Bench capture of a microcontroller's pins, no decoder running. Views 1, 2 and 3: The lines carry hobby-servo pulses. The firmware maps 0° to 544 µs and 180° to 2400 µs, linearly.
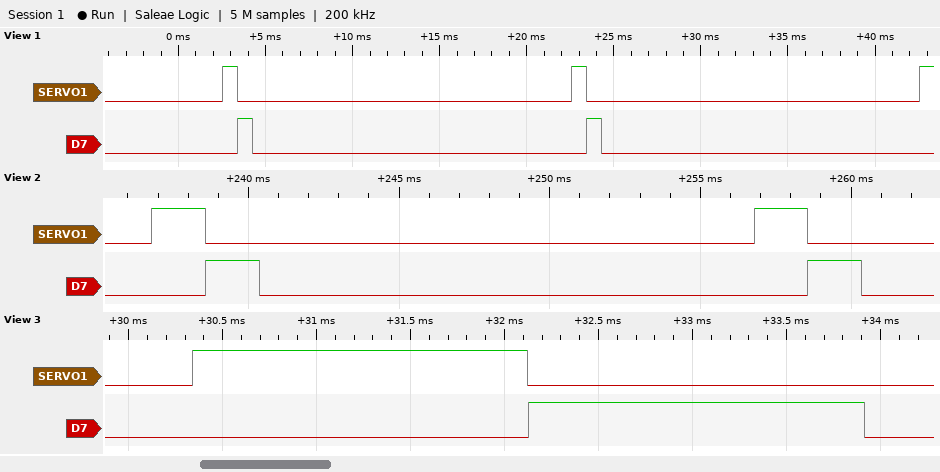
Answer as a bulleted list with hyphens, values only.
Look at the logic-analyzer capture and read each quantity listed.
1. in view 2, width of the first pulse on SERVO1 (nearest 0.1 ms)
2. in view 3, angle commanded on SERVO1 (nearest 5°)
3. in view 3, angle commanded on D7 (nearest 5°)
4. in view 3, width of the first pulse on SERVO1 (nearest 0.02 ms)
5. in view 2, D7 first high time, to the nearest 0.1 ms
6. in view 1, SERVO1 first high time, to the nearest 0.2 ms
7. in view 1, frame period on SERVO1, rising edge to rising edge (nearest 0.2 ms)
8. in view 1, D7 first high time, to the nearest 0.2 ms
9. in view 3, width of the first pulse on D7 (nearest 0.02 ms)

- 1.8 ms
- 120°
- 120°
- 1.78 ms
- 1.8 ms
- 0.8 ms
- 20.0 ms
- 0.8 ms
- 1.78 ms
